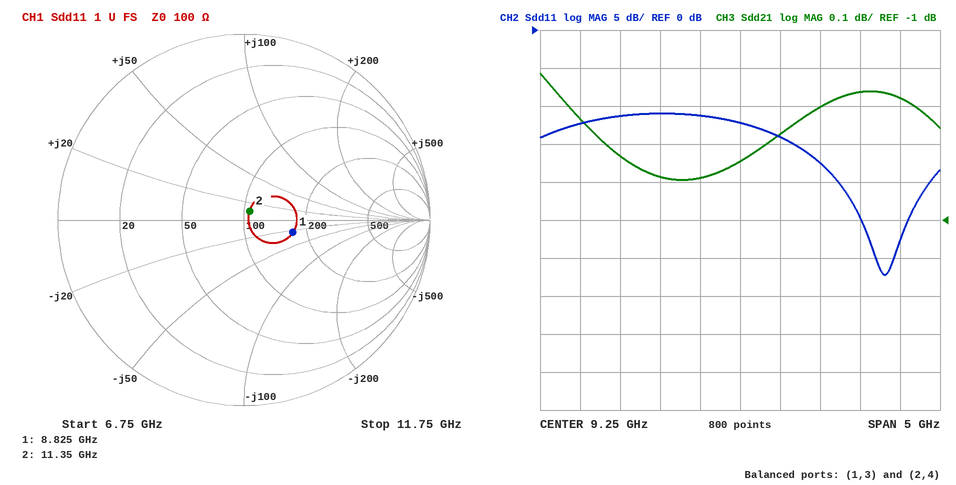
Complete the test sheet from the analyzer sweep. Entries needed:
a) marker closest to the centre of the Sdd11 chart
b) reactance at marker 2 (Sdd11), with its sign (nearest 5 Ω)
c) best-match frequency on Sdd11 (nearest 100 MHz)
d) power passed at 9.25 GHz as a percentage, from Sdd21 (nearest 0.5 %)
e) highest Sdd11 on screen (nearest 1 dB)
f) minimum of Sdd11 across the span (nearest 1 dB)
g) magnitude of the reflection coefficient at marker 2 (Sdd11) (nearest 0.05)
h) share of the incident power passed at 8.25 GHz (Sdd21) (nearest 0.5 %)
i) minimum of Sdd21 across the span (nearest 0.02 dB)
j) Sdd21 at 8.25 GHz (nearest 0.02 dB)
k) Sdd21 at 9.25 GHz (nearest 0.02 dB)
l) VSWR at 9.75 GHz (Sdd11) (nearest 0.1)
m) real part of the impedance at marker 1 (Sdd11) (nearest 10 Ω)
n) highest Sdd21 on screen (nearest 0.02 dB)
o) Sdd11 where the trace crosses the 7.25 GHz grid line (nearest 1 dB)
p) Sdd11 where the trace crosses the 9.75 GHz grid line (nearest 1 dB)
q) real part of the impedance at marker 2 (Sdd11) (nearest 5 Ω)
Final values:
marker 2
+10 Ω
11.1 GHz
82.5 %
-11 dB
-32 dB
0.05
81.5 %
-0.90 dB
-0.88 dB
-0.84 dB
1.5
170 Ω
-0.62 dB
-12 dB
-14 dB
105 Ω
